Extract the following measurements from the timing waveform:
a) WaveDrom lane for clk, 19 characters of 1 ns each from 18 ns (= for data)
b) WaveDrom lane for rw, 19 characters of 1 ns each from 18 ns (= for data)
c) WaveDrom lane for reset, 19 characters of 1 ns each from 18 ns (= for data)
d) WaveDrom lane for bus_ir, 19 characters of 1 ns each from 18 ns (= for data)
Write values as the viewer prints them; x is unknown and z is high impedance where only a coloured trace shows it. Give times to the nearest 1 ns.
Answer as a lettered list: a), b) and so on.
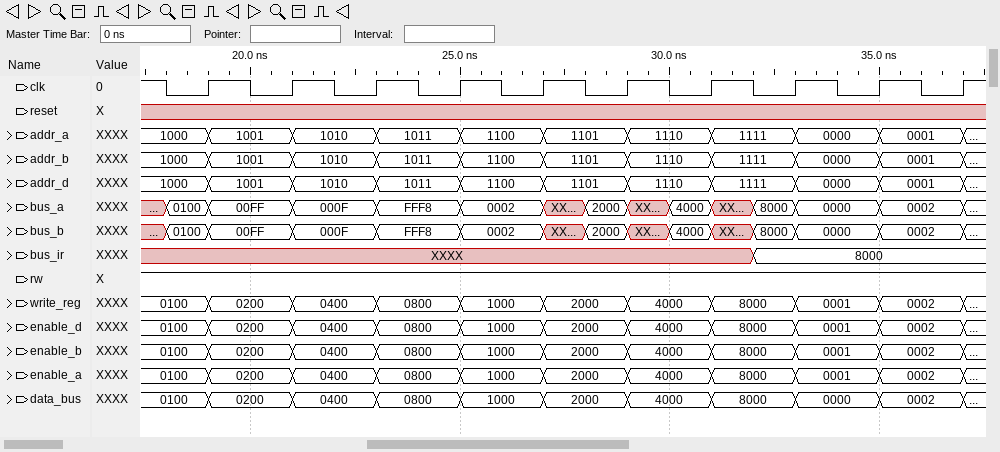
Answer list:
a) {name: 'clk', wave: '0101010101010101010'}
b) {name: 'rw', wave: '1..................'}
c) {name: 'reset', wave: 'x..................'}
d) {name: 'bus_ir', wave: 'x.............=....', data: '8000'}
